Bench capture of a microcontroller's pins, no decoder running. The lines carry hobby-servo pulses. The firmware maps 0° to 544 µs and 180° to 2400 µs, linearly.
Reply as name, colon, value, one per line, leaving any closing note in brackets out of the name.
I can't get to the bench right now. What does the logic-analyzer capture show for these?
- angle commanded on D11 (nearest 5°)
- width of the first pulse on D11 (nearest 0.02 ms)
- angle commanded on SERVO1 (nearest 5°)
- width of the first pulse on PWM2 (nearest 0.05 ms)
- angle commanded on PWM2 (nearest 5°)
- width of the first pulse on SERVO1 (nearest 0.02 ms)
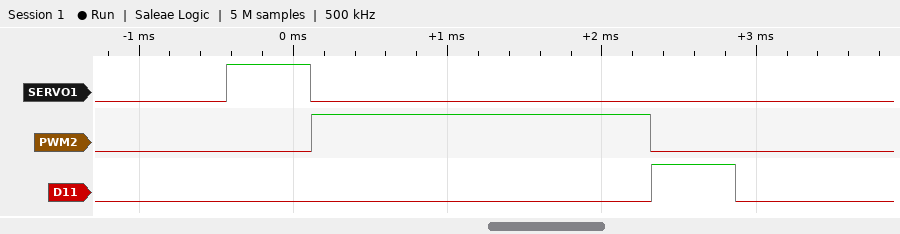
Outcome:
angle commanded on D11: 0°
width of the first pulse on D11: 0.54 ms
angle commanded on SERVO1: 0°
width of the first pulse on PWM2: 2.20 ms
angle commanded on PWM2: 160°
width of the first pulse on SERVO1: 0.54 ms
